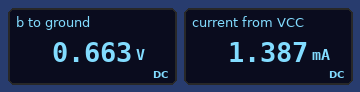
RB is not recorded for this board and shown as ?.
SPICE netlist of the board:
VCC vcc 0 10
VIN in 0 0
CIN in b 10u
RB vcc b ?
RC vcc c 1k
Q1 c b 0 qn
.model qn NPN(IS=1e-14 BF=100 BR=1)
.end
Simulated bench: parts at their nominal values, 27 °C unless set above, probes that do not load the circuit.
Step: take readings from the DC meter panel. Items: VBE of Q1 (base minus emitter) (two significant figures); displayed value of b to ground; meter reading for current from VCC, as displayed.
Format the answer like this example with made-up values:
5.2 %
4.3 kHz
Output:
660 mV
0.663 V
1.387 mA
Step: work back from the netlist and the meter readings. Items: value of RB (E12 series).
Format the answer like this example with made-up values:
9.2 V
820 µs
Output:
680 kΩ
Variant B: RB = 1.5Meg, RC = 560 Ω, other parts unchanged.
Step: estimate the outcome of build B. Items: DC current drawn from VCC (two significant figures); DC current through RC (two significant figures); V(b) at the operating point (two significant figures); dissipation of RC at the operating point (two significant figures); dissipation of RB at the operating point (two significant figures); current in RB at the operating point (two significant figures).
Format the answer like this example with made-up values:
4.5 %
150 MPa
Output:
630 µA
620 µA
640 mV
220 µW
58 µW
6.2 µA
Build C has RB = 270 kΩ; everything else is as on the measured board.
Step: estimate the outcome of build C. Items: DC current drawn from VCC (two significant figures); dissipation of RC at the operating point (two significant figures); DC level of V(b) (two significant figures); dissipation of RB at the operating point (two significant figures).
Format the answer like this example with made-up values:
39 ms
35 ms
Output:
3.5 mA
12 mW
690 mV
320 µW
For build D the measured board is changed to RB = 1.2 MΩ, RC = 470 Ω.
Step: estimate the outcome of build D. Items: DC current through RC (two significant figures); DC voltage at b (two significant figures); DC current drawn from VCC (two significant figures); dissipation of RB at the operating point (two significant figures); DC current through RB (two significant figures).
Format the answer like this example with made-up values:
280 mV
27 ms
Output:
780 µA
650 mV
790 µA
73 µW
7.8 µA
